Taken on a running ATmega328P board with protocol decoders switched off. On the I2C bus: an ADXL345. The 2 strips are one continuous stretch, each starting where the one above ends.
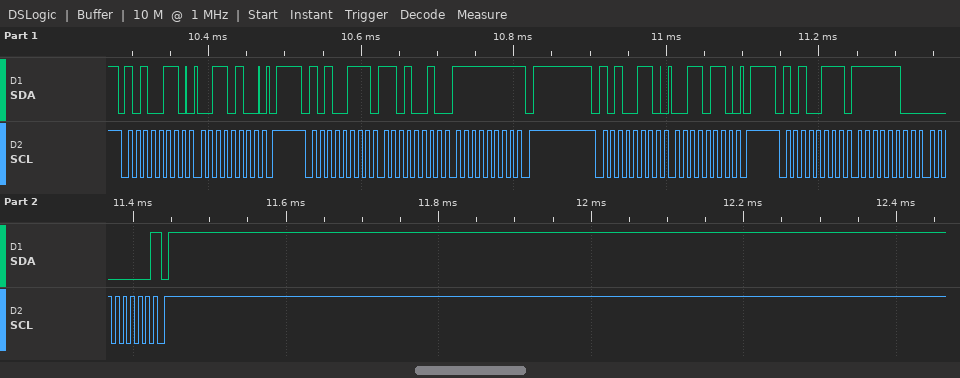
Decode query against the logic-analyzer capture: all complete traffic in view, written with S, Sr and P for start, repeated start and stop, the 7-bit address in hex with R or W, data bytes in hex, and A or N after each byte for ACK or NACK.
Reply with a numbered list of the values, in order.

1. S 53W A 34 A P S 53R A D2 A FF N P S 53W A 36 A P S 53R A FC A 00 N P
